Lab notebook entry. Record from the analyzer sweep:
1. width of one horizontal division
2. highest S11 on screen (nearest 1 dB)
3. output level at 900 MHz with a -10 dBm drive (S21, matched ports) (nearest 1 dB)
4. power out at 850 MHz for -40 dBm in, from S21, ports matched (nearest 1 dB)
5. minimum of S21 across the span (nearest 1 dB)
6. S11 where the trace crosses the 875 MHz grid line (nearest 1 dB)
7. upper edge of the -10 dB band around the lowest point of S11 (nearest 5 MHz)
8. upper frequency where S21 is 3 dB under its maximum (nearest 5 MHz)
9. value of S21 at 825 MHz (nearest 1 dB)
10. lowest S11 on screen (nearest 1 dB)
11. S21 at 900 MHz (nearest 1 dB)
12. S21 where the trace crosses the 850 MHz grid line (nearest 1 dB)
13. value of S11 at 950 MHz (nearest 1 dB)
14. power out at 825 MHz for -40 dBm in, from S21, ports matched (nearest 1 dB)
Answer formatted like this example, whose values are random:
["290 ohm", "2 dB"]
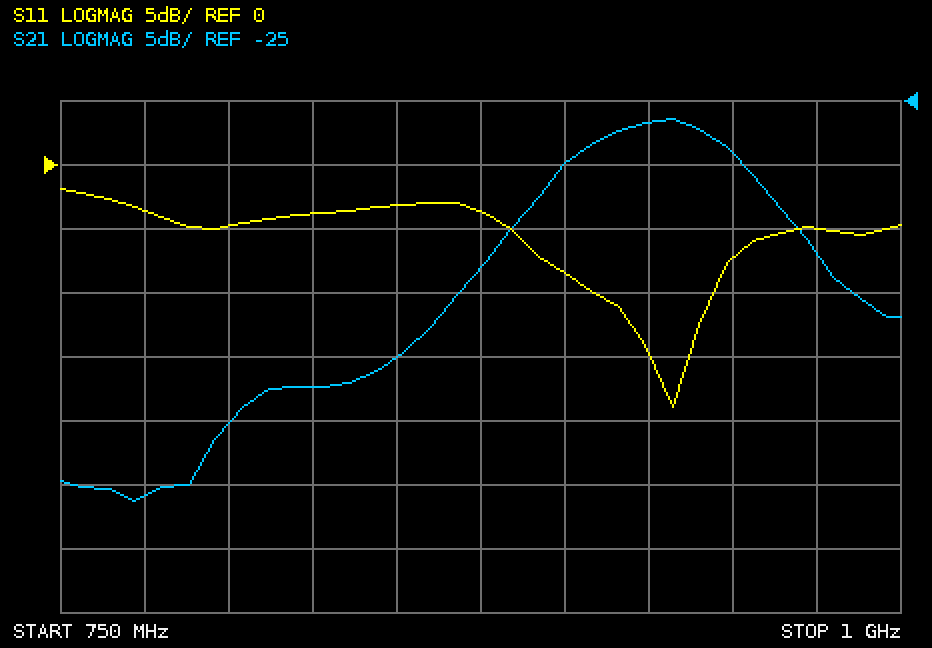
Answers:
["25 MHz", "-2 dB", "-40 dBm", "-85 dBm", "-56 dB", "-4 dB", "945 MHz", "950 MHz", "-47 dB", "-19 dB", "-30 dB", "-45 dB", "-7 dB", "-87 dBm"]
